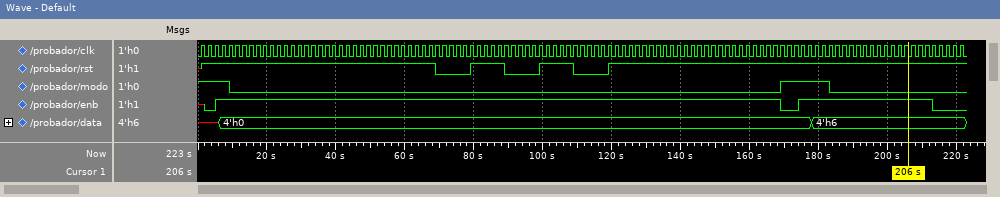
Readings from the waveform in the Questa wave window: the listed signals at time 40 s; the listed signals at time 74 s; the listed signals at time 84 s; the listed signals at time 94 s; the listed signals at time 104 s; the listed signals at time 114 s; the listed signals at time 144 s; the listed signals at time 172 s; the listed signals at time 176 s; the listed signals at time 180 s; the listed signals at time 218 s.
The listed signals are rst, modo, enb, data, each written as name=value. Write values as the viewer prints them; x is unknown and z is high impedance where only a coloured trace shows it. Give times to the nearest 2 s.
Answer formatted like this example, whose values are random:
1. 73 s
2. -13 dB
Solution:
1. rst=1, modo=0, enb=1, data=4'h0
2. rst=0, modo=0, enb=1, data=4'h0
3. rst=1, modo=0, enb=1, data=4'h0
4. rst=0, modo=0, enb=1, data=4'h0
5. rst=1, modo=0, enb=1, data=4'h0
6. rst=0, modo=0, enb=1, data=4'h0
7. rst=1, modo=0, enb=1, data=4'h0
8. rst=1, modo=1, enb=0, data=4'h0
9. rst=1, modo=1, enb=1, data=4'h0
10. rst=1, modo=1, enb=1, data=4'h6
11. rst=1, modo=0, enb=0, data=4'h6
